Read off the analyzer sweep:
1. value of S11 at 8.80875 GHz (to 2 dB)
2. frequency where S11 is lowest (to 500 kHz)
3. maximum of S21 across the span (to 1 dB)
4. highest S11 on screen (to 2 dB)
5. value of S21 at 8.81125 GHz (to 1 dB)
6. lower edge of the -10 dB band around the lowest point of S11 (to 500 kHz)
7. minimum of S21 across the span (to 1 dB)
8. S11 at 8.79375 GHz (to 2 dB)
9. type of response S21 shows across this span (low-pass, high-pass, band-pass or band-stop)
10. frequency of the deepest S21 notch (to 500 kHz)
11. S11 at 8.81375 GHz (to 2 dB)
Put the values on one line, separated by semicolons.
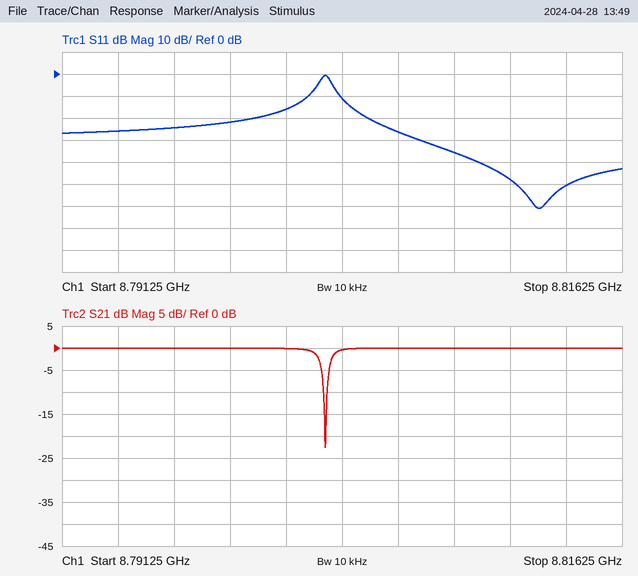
-36 dB; 8.8125 GHz; 0 dB; 0 dB; 0 dB; 8.8035 GHz; -23 dB; -26 dB; band-stop; 8.8030 GHz; -50 dB
